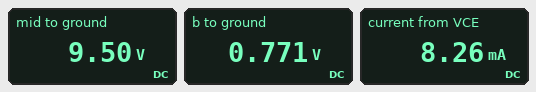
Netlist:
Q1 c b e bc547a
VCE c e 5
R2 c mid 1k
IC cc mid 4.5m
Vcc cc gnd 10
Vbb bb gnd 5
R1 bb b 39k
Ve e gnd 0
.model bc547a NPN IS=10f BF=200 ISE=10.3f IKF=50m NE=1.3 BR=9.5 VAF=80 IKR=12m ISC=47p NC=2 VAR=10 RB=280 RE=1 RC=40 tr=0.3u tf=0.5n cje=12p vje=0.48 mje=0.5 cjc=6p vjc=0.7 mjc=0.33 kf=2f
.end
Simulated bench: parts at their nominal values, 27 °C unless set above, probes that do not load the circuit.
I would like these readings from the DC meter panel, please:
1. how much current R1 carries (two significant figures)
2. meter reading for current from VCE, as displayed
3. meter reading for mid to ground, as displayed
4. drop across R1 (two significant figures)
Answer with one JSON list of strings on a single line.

["110 µA", "8.26 mA", "9.50 V", "4.2 V"]
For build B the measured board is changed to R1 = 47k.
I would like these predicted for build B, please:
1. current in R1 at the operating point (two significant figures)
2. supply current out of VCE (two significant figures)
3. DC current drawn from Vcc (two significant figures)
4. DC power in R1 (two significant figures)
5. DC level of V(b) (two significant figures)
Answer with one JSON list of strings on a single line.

["90 µA", "6.4 mA", "4.5 mA", "380 µW", "760 mV"]
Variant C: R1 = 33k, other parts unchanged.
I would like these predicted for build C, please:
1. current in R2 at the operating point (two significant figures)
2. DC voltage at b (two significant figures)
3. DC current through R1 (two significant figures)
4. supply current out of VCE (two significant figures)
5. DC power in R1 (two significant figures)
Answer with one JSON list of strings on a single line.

["4.5 mA", "780 mV", "130 µA", "10 mA", "540 µW"]
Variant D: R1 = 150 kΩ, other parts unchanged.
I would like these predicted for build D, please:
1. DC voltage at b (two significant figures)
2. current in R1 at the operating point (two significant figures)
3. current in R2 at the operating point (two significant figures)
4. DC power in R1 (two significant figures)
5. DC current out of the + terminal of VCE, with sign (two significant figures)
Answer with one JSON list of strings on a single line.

["700 mV", "29 µA", "4.5 mA", "120 µW", "-840 µA"]
